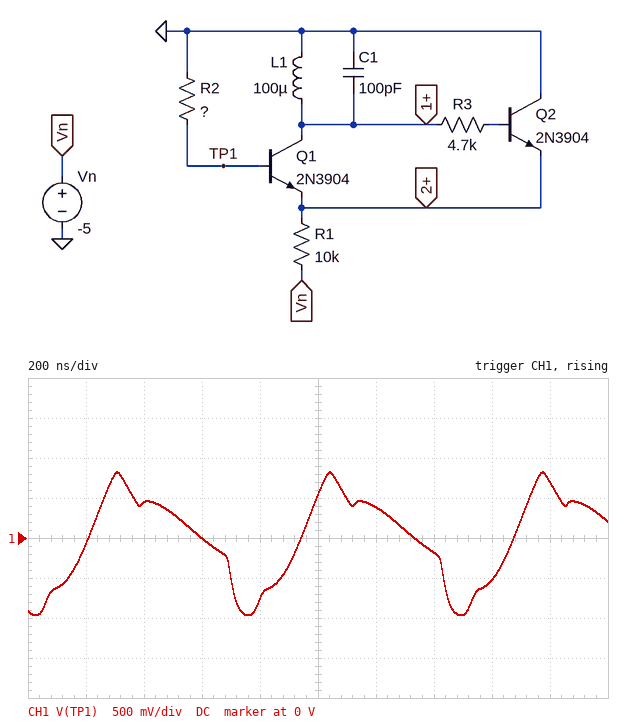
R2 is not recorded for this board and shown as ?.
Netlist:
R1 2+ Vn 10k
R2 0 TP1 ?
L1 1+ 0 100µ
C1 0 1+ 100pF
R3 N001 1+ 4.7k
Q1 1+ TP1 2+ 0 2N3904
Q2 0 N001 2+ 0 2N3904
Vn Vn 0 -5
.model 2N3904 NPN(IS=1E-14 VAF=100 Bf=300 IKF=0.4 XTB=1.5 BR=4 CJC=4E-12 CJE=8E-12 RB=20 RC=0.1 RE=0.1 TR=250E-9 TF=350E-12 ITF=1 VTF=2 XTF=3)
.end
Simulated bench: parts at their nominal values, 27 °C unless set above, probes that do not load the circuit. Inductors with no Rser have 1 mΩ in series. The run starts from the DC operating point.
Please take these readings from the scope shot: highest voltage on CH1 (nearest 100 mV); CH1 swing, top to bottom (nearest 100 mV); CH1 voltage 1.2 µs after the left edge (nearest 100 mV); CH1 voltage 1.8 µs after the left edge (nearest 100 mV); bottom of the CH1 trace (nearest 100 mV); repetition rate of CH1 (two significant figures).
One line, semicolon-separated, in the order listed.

800 mV; 1.8 V; 400 mV; 700 mV; -1.0 V; 1.4 MHz
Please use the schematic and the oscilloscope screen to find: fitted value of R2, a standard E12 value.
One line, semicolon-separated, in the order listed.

12 kΩ
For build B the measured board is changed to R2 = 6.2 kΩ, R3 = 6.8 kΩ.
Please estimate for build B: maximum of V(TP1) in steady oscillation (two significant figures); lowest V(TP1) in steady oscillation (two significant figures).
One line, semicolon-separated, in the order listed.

990 mV; -780 mV
